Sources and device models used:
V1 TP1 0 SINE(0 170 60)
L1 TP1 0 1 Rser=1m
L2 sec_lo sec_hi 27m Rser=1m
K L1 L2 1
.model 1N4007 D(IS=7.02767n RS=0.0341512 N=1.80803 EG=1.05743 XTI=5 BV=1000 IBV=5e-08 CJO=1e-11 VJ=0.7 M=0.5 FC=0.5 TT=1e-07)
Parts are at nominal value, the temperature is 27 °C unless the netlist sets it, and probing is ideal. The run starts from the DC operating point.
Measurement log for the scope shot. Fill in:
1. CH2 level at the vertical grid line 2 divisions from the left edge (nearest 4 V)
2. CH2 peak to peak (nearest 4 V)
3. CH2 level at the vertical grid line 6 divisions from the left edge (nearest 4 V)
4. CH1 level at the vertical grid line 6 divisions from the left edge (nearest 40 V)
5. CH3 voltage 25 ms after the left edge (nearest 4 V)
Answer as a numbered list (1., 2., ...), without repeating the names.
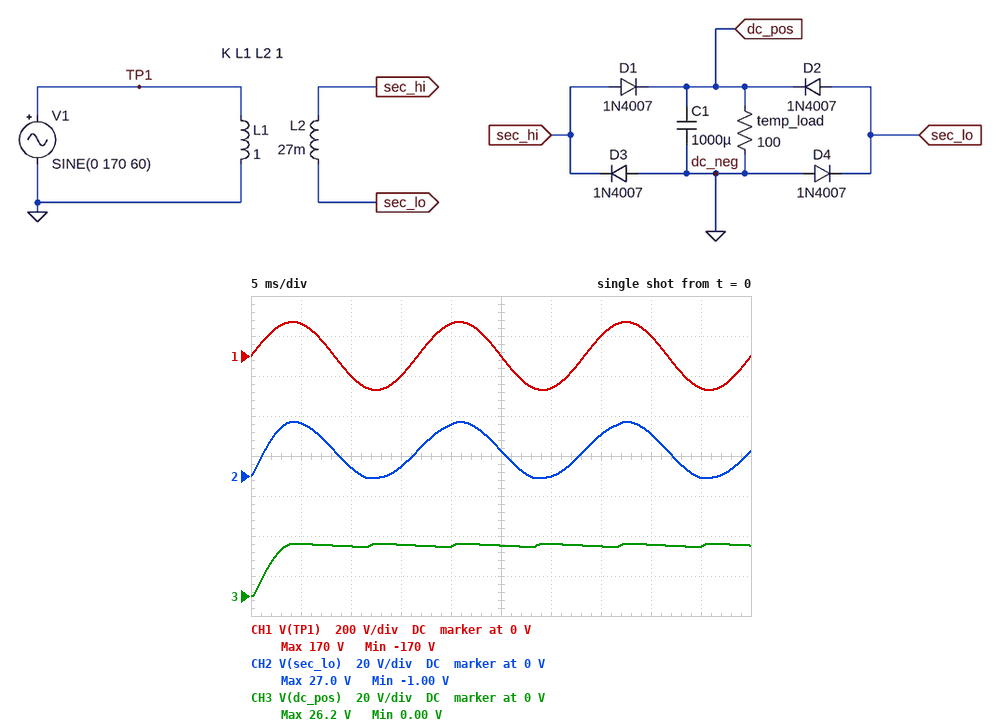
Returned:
1. 4 V
2. 28 V
3. 0 V
4. -160 V
5. 24 V
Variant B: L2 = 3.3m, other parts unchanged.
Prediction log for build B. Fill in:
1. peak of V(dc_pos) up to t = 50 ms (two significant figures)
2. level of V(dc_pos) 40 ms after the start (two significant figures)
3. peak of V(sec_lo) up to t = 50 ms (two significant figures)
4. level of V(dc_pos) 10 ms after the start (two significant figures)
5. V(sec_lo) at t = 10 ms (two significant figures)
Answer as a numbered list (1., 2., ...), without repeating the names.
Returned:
1. 8.1 V
2. 8.0 V
3. 8.9 V
4. 7.7 V
5. 980 mV
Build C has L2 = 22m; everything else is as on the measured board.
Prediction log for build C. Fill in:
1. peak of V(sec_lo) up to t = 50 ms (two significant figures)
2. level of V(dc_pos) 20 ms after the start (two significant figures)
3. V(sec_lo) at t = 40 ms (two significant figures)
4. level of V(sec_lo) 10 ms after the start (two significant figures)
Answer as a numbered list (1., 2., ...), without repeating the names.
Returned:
1. 24 V
2. 22 V
3. 19 V
4. 3.7 V
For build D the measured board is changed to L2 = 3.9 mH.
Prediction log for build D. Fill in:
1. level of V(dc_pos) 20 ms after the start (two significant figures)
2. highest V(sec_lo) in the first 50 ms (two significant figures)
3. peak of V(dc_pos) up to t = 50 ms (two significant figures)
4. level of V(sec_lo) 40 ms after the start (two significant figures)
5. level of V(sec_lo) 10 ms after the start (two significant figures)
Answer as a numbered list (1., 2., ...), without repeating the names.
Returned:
1. 8.4 V
2. 9.8 V
3. 9.0 V
4. 7.5 V
5. 1.1 V
